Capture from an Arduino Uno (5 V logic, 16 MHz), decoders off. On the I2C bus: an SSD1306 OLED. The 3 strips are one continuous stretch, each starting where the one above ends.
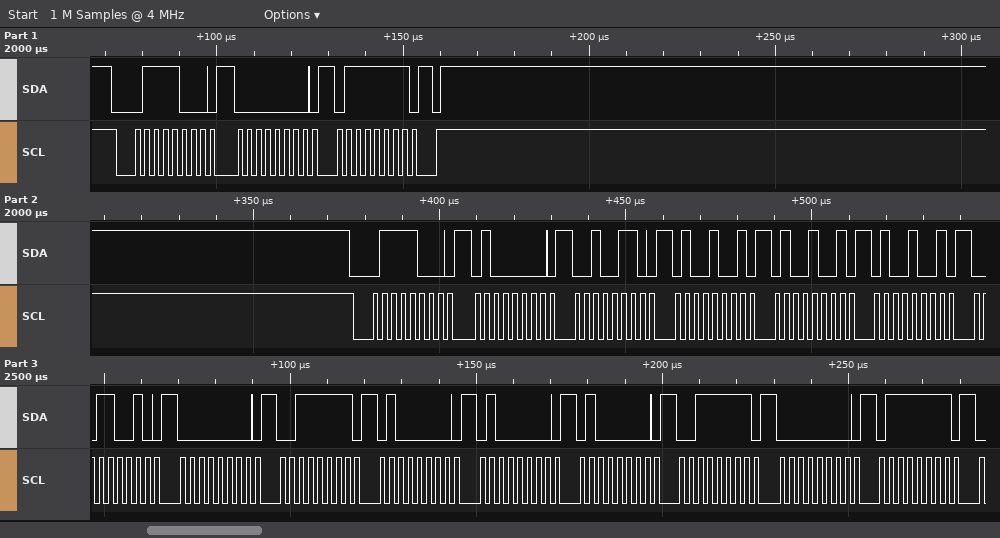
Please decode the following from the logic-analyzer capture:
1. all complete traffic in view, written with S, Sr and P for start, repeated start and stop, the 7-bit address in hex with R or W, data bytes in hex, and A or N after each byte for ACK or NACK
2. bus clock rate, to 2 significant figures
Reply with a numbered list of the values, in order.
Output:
1. S 3CW A 00 A 7F A P S 3CW A 40 A 26 A 49 A 49 A 49 A 32 A 00 A 3F A 40 A 40 A 40 A 3F A 00 A 7F A
2. 400 kHz
